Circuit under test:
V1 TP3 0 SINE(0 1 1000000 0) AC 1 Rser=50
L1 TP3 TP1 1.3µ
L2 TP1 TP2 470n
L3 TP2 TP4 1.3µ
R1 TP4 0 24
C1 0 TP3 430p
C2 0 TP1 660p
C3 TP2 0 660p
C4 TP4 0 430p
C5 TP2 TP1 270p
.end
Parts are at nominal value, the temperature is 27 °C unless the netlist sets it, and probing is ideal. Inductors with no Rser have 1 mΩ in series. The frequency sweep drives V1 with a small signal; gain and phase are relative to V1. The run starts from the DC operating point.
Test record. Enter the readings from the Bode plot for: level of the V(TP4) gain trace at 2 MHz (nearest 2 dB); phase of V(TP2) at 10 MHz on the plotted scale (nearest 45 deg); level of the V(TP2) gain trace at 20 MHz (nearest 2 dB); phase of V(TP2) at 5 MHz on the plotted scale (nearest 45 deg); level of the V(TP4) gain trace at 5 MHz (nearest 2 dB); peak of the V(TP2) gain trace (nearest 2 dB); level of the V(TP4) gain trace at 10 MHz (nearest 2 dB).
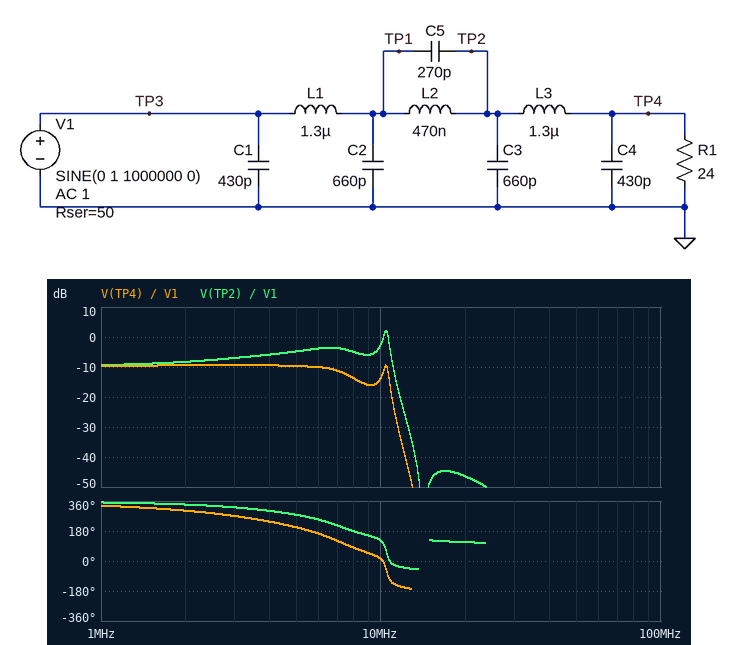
-10 dB
135 deg
-46 dB
270 deg
-10 dB
2 dB
-14 dB
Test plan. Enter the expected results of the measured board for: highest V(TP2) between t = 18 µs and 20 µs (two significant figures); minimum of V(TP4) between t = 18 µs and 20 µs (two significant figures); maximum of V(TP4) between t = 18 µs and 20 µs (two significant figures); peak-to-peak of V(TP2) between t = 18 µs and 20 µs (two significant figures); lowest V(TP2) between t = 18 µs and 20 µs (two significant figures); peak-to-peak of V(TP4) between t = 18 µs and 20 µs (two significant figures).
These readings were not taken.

340 mV
-330 mV
330 mV
680 mV
-340 mV
660 mV
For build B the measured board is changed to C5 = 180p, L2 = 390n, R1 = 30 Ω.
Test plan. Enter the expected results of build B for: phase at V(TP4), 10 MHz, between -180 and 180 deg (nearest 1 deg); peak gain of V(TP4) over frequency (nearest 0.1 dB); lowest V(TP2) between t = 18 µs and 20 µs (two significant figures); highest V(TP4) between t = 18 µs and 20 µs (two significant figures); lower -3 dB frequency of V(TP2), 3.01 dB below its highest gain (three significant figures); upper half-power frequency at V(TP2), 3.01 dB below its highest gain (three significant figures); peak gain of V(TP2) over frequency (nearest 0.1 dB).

31 deg
-8.2 dB
-380 mV
380 mV
12.1 MHz
12.4 MHz
3.9 dB
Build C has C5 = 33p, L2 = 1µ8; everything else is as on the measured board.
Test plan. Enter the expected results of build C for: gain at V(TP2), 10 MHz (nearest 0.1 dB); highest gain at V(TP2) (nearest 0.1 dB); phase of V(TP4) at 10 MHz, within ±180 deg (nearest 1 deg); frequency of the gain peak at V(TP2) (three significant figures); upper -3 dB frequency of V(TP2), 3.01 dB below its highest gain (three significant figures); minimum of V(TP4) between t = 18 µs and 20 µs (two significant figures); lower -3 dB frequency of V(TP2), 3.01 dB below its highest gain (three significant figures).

-15.1 dB
-1.0 dB
-120 deg
8.01 MHz
8.85 MHz
-330 mV
5.73 MHz
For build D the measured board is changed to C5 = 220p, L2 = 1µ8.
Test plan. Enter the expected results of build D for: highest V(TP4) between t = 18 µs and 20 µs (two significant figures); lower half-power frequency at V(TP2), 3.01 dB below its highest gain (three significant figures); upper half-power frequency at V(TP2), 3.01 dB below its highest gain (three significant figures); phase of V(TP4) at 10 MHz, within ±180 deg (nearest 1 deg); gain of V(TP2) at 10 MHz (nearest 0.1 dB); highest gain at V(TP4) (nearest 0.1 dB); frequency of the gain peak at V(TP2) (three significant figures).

330 mV
2.16 MHz
6.74 MHz
49 deg
-26.2 dB
-9.7 dB
5.98 MHz
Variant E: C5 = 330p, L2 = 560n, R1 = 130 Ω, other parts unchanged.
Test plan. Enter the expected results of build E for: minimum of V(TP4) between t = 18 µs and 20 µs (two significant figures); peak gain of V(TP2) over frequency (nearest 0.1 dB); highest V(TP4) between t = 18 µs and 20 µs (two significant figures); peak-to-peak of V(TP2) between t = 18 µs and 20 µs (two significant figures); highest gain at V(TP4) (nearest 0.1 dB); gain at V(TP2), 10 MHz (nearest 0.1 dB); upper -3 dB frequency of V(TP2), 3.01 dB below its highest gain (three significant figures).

-690 mV
-1.0 dB
690 mV
1.4 V
-1.9 dB
-9.1 dB
9.77 MHz
